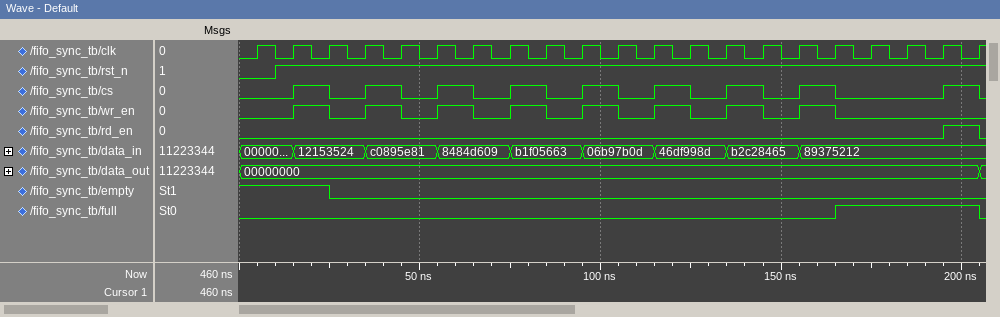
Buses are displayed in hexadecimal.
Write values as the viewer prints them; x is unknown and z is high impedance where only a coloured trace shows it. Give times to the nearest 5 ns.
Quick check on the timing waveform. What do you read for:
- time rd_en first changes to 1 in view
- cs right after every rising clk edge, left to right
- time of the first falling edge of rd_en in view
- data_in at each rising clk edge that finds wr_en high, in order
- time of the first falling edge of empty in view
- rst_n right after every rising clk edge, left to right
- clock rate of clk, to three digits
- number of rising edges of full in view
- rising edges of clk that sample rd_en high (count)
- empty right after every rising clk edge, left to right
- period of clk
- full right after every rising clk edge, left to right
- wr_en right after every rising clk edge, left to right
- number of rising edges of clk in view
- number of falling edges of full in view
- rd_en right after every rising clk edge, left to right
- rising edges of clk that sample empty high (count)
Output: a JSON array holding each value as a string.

["195 ns", "0 1 0 1 0 1 0 1 0 1 0 1 0 1 0 1 0 0 0 1 0", "205 ns", "12153524, c0895e81, 8484d609, b1f05663, 06b97b0d, 46df998d, b2c28465, 89375212", "25 ns", "0 1 1 1 1 1 1 1 1 1 1 1 1 1 1 1 1 1 1 1 1", "100 MHz", "1", "1", "1 1 0 0 0 0 0 0 0 0 0 0 0 0 0 0 0 0 0 0 0", "10 ns", "0 0 0 0 0 0 0 0 0 0 0 0 0 0 0 0 1 1 1 1 0", "0 1 0 1 0 1 0 1 0 1 0 1 0 1 0 1 0 0 0 0 0", "21", "1", "0 0 0 0 0 0 0 0 0 0 0 0 0 0 0 0 0 0 0 1 0", "3"]
